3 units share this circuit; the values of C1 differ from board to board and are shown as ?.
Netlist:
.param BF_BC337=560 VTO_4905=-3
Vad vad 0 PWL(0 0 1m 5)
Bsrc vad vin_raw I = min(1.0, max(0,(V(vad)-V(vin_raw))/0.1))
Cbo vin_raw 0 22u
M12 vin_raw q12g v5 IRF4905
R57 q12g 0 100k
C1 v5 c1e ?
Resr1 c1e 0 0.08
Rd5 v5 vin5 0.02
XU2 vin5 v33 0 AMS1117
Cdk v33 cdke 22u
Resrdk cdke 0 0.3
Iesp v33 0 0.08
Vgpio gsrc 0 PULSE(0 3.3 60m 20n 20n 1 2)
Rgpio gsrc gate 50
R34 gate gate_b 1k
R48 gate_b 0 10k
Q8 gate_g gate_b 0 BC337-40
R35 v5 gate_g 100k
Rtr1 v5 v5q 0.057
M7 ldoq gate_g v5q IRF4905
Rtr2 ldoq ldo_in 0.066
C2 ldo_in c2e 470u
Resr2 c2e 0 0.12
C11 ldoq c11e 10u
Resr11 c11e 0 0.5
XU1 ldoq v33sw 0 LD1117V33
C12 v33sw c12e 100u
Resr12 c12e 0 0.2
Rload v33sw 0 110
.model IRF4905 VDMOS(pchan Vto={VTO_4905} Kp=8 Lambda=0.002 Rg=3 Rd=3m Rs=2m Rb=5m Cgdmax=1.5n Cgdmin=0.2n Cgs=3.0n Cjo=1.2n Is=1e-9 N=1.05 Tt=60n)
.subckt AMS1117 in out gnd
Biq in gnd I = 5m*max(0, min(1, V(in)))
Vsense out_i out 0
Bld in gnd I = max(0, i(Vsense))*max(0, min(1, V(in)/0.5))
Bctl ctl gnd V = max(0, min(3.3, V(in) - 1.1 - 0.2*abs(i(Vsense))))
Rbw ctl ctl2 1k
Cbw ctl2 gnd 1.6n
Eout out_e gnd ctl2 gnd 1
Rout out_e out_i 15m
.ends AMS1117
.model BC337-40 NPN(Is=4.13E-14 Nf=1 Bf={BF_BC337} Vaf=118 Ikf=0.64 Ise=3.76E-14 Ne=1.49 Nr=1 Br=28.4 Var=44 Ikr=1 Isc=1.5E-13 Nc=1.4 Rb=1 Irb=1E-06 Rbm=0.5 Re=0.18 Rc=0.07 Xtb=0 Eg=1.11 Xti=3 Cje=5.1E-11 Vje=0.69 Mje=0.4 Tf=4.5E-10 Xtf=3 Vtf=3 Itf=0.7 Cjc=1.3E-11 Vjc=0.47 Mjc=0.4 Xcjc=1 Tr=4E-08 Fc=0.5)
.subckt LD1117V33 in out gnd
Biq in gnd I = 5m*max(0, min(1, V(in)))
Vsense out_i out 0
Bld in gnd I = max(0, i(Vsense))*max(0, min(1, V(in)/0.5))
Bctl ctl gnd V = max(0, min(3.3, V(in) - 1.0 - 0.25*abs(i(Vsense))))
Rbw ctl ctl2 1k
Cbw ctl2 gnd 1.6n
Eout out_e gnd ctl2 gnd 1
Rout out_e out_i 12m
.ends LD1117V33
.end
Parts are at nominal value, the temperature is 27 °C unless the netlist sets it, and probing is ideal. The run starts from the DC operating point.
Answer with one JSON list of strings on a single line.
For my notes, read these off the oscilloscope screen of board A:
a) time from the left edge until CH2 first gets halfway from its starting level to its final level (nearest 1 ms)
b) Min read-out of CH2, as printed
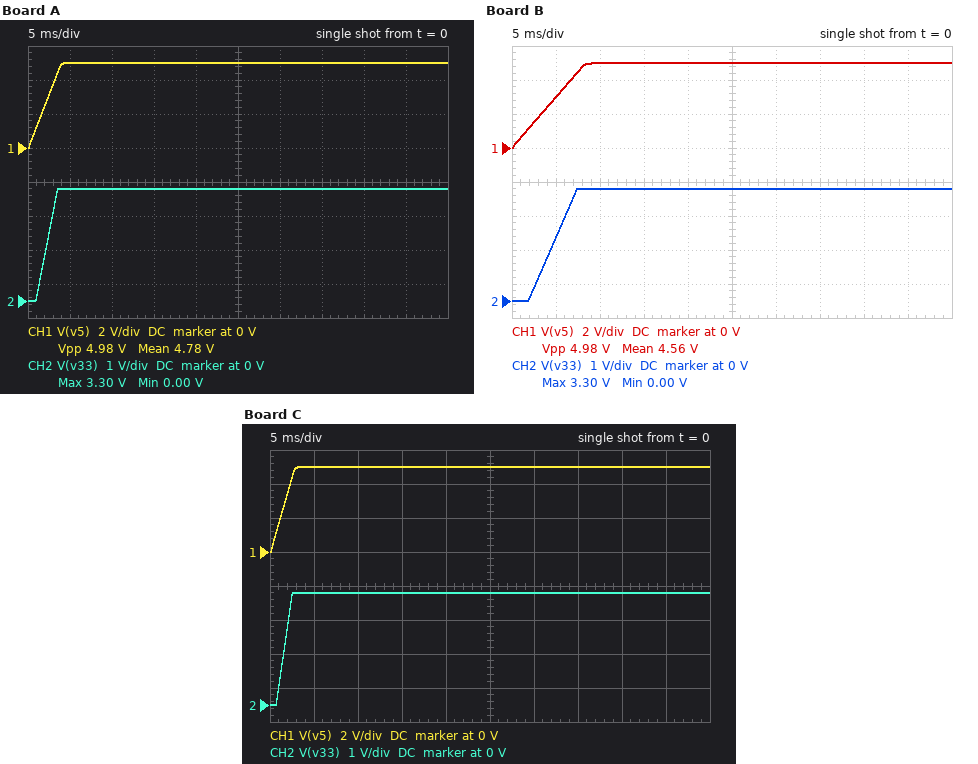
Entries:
["2 ms", "0.00 V"]
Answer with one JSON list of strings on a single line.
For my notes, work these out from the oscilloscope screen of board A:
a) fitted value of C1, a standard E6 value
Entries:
["680 µF"]
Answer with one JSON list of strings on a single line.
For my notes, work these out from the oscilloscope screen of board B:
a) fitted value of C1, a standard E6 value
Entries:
["1.5 mF"]
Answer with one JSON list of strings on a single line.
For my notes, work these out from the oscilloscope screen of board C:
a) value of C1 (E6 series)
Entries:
["470 µF"]
